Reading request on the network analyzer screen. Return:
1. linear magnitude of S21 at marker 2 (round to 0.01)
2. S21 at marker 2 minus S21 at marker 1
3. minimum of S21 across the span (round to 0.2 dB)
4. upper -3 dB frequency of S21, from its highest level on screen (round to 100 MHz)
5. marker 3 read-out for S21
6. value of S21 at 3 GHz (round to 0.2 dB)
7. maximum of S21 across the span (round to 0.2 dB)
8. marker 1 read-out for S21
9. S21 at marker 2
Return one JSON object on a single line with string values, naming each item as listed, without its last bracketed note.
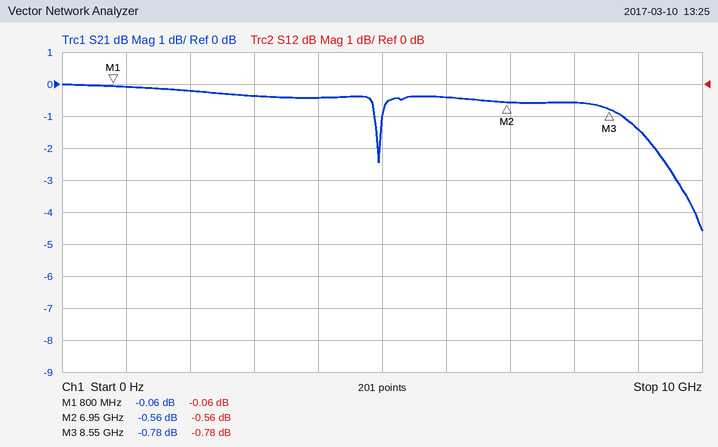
{"linear magnitude of S21 at marker 2": "0.94", "S21 at marker 2 minus S21 at marker 1": "-0.50 dB", "minimum of S21 across the span": "-4.6 dB", "upper -3 dB frequency of S21, from its highest level on screen": "9.6 GHz", "marker 3 read-out for S21": "-0.78 dB", "value of S21 at 3 GHz": "-0.4 dB", "maximum of S21 across the span": "0.0 dB", "marker 1 read-out for S21": "-0.06 dB", "S21 at marker 2": "-0.56 dB"}
